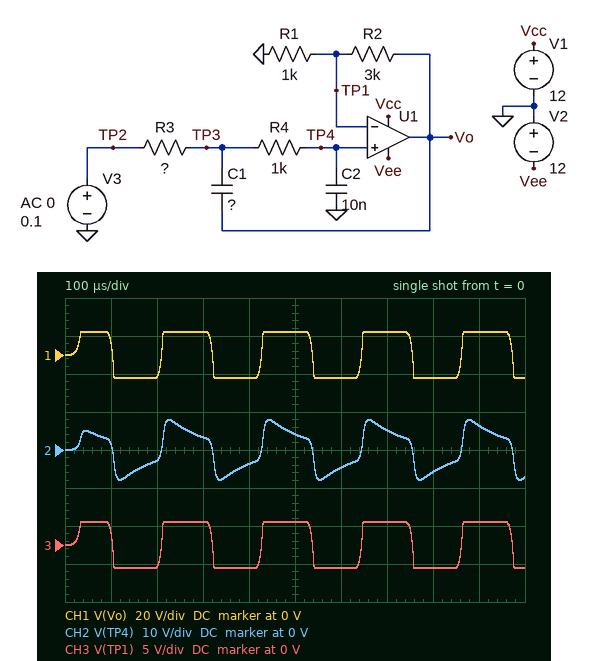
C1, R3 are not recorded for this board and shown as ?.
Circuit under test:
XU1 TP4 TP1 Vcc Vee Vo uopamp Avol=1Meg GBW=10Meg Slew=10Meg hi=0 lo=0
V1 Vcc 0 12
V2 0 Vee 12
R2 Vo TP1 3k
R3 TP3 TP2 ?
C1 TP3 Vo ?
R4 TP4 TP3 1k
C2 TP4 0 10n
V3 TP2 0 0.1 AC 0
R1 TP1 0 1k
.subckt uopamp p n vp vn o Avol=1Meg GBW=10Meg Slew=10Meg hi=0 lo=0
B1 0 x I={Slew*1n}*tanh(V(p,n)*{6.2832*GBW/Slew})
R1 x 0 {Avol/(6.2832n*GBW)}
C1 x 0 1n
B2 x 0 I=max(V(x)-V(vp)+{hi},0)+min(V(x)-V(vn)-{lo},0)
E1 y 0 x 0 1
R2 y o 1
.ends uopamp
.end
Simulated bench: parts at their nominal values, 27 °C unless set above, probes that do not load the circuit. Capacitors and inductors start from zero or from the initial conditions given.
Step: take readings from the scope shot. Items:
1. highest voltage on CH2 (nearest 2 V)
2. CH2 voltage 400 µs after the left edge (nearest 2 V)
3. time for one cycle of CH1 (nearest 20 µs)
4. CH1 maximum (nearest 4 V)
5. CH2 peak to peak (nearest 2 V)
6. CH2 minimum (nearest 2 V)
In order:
8 V
-4 V
220 µs
12 V
16 V
-8 V
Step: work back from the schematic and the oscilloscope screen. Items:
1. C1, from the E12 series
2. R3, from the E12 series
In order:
12 nF
3.3 kΩ
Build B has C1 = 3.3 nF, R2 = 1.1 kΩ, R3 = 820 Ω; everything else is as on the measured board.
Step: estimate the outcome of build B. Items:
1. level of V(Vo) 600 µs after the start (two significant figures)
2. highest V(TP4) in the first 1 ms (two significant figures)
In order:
210 mV
100 mV
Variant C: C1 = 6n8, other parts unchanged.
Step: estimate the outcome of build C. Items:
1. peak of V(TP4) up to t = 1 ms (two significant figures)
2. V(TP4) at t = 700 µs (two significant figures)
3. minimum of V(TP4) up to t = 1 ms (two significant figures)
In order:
5.1 V
3.0 V
-5.1 V
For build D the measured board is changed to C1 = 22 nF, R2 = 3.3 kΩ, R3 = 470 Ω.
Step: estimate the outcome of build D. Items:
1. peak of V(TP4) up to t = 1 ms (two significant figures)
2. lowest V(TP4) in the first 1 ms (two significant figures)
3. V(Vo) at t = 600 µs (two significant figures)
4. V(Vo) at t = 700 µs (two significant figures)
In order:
6.4 V
-6.3 V
12 V
-12 V
